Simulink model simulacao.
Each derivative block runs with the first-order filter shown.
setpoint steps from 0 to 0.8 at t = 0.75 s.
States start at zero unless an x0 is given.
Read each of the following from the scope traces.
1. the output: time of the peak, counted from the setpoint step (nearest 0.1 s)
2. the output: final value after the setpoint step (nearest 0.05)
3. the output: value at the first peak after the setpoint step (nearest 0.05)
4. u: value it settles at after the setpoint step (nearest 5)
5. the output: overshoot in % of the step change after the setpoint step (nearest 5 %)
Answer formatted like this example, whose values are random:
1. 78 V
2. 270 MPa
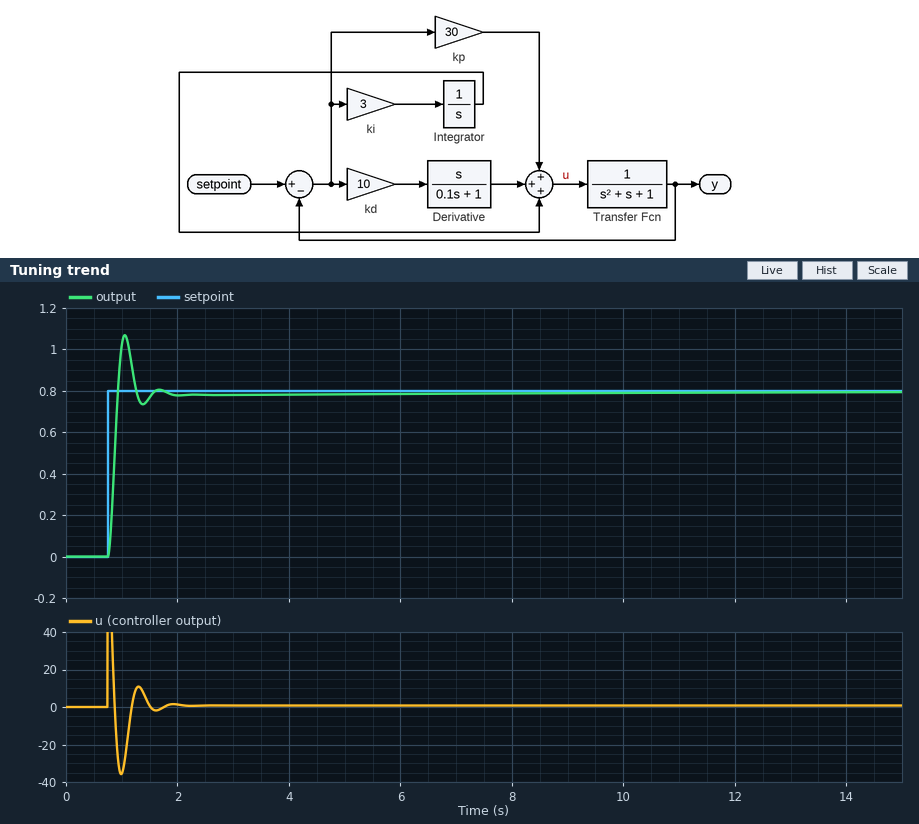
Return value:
1. 0.3 s
2. 0.80
3. 1.05
4. 0
5. 35 %
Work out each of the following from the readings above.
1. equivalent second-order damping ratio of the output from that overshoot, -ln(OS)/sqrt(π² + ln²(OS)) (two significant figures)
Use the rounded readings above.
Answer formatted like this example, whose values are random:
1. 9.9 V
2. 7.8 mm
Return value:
1. 0.32
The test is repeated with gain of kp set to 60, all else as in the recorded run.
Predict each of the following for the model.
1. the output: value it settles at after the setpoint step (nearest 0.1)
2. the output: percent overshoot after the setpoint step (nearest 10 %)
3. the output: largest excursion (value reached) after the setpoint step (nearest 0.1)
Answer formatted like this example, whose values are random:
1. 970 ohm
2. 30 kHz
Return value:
1. 0.8
2. 50 %
3. 1.2
